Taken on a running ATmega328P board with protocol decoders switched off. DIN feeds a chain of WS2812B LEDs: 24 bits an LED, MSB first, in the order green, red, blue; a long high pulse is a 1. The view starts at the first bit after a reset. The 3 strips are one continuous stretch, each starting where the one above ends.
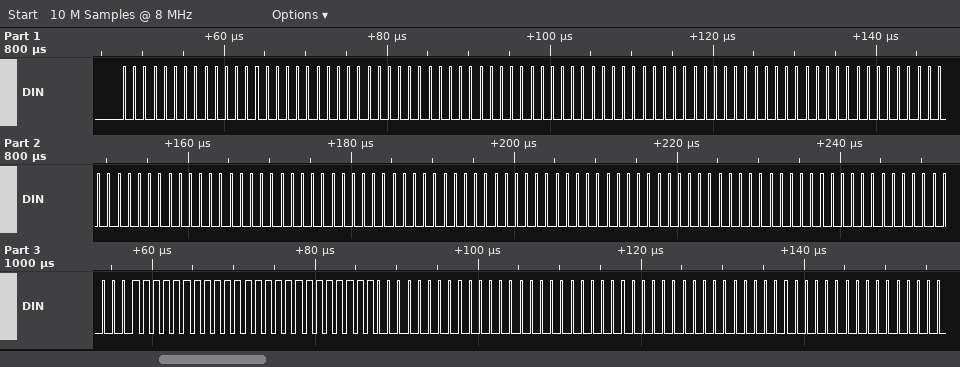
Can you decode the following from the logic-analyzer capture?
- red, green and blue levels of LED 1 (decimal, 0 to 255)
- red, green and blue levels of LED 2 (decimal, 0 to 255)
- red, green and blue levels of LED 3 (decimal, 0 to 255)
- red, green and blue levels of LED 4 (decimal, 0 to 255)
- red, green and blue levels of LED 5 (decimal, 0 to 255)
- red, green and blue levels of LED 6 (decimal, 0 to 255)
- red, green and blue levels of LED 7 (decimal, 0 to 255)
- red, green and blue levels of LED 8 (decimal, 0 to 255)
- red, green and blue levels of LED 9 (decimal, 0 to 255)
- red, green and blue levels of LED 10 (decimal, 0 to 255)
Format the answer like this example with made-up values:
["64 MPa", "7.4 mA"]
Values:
["0, 0, 0", "0, 0, 0", "0, 0, 0", "0, 0, 0", "0, 0, 0", "0, 0, 0", "0, 0, 0", "255, 255, 255", "0, 0, 0", "0, 0, 0"]
